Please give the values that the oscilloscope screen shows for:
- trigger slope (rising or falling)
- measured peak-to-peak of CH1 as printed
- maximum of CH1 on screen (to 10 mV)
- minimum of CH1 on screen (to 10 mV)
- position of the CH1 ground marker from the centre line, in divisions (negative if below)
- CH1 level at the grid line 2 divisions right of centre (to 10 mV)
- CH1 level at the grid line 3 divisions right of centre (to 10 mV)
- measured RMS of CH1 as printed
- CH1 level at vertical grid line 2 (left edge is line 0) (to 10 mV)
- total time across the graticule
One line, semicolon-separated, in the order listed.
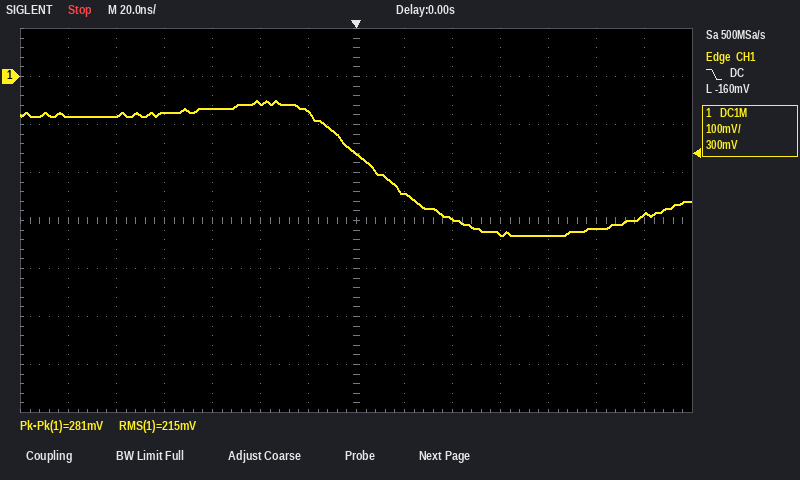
falling; 281 mV; -50 mV; -330 mV; +3.0 div; -300 mV; -330 mV; 215 mV; -80 mV; 280 ns
